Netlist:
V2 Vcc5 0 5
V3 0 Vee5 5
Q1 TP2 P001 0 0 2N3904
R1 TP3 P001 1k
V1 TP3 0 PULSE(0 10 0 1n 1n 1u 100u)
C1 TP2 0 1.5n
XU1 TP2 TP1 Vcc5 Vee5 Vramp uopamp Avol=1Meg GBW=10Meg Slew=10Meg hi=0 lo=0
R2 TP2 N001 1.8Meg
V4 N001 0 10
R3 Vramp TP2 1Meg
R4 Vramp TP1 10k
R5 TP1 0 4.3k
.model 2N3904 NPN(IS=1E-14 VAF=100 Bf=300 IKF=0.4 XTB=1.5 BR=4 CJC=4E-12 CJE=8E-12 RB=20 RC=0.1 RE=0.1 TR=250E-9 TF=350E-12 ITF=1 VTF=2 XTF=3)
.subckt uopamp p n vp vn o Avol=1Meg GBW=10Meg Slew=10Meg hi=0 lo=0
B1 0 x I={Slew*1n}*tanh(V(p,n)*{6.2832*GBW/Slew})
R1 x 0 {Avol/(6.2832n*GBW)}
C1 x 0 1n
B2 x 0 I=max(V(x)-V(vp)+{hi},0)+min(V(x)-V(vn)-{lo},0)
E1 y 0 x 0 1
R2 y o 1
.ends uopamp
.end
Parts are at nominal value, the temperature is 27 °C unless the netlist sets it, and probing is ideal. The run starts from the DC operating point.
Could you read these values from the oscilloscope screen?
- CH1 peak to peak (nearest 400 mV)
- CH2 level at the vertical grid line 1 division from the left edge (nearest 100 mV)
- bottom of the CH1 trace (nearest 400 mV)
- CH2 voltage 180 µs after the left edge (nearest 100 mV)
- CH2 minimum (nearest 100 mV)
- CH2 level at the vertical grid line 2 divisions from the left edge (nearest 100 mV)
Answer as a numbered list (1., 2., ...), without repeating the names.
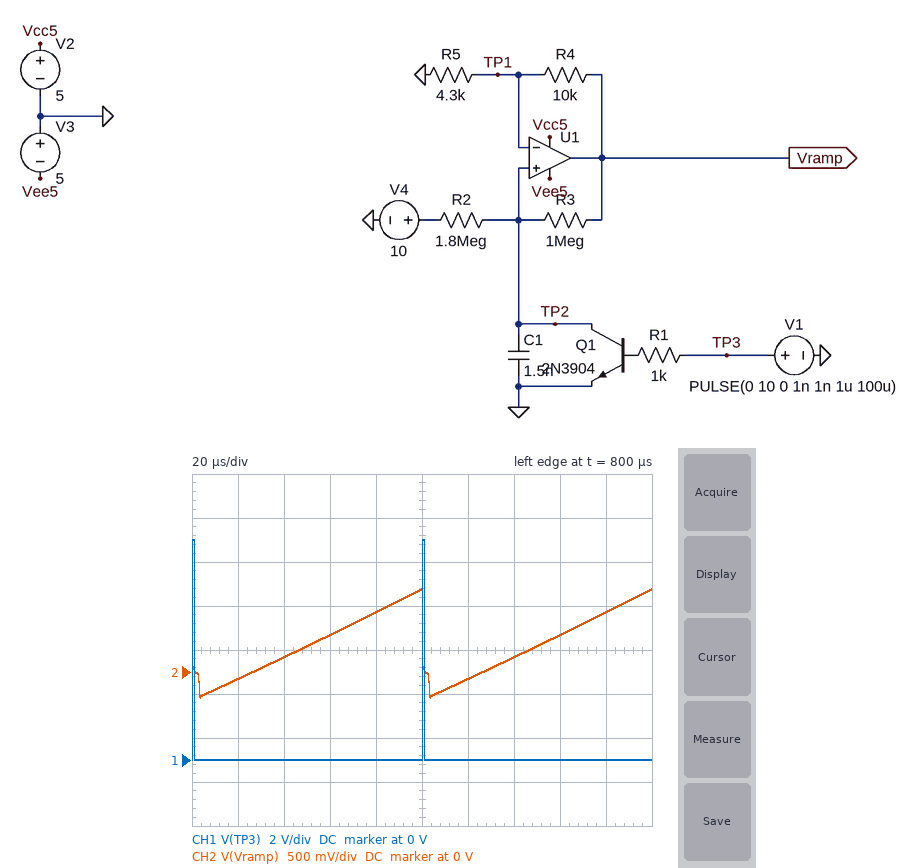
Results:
1. 10.0 V
2. -100 mV
3. 0 V
4. 700 mV
5. -300 mV
6. 200 mV
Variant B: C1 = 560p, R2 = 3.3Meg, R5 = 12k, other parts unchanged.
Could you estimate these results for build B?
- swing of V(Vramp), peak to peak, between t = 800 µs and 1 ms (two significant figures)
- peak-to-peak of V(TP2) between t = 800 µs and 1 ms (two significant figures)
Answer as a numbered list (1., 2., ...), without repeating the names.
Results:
1. 970 mV
2. 530 mV
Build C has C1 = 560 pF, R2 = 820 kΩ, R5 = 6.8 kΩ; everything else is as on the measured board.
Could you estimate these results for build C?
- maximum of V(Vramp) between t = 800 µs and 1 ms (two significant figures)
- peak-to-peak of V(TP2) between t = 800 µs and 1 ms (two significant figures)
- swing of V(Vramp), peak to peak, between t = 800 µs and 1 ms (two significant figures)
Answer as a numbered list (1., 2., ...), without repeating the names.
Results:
1. 4.9 V
2. 2.1 V
3. 5.3 V
